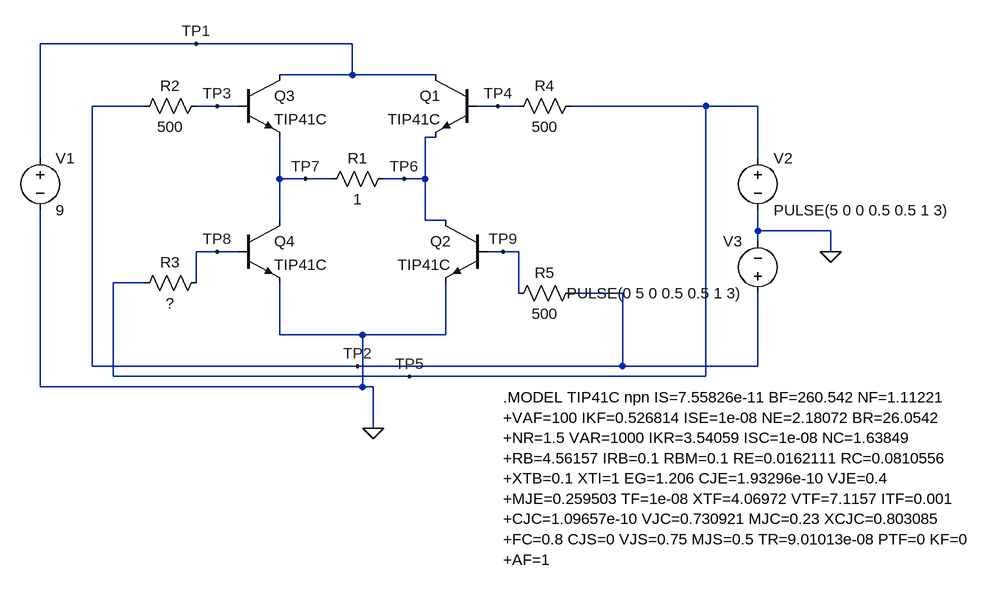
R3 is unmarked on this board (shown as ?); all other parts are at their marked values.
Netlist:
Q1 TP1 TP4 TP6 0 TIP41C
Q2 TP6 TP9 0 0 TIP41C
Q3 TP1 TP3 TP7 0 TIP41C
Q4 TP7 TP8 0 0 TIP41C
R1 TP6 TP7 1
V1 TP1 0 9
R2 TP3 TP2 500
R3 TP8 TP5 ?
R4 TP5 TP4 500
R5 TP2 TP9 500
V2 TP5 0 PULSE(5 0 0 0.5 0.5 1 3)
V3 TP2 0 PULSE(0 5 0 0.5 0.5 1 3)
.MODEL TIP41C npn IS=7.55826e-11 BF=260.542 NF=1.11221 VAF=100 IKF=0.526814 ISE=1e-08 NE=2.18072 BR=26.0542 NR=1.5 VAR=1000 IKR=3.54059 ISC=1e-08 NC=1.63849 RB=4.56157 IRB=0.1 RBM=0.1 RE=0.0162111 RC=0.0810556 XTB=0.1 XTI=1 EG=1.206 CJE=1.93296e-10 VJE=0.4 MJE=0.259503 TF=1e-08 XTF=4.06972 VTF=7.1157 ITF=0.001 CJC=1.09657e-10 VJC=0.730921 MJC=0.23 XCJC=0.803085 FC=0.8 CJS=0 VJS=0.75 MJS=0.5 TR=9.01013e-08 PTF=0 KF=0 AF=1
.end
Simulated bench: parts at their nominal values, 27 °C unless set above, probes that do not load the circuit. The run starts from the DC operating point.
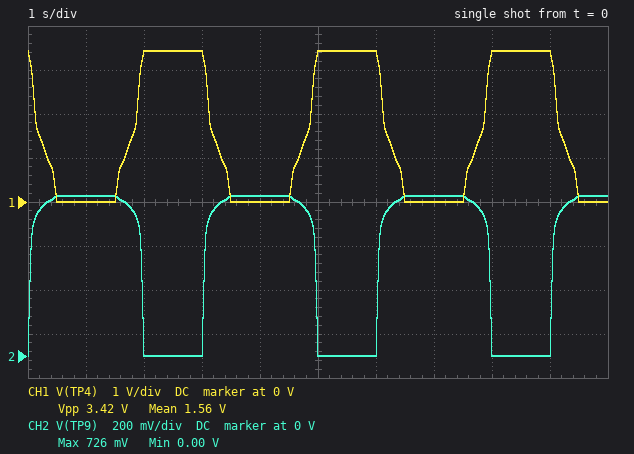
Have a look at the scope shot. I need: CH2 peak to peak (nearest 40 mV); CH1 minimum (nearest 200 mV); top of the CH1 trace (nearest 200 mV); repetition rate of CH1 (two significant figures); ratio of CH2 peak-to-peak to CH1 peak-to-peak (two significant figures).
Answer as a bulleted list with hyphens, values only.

- 720 mV
- 0 V
- 3.4 V
- 330 mHz
- 0.21
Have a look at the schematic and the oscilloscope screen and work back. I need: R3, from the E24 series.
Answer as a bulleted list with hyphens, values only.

- 1.3 kΩ
